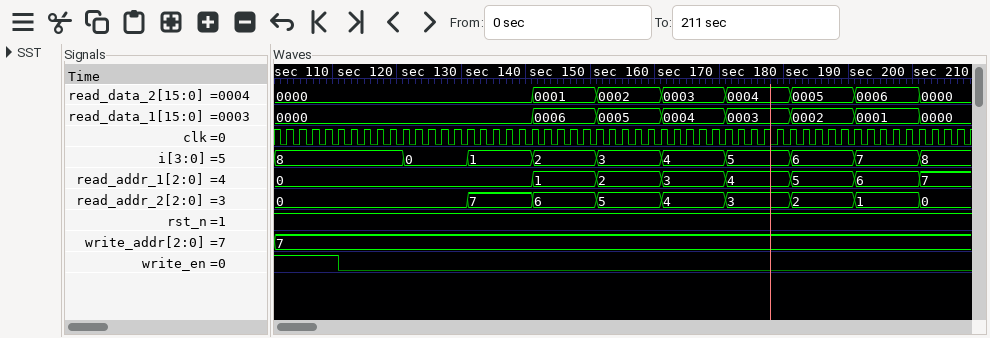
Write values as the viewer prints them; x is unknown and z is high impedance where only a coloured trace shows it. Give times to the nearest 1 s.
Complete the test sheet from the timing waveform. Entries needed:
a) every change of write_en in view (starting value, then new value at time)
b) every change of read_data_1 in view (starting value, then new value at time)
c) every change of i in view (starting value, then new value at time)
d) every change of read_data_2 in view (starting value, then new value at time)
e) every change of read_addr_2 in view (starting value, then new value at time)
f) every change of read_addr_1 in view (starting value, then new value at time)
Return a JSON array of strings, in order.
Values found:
["1, 0 at 111 s", "0000, 0006 at 141 s, 0005 at 151 s, 0004 at 161 s, 0003 at 171 s, 0002 at 181 s, 0001 at 191 s, 0000 at 201 s", "8, 0 at 121 s, 1 at 131 s, 2 at 141 s, 3 at 151 s, 4 at 161 s, 5 at 171 s, 6 at 181 s, 7 at 191 s, 8 at 201 s", "0000, 0001 at 141 s, 0002 at 151 s, 0003 at 161 s, 0004 at 171 s, 0005 at 181 s, 0006 at 191 s, 0000 at 201 s", "0, 7 at 131 s, 6 at 141 s, 5 at 151 s, 4 at 161 s, 3 at 171 s, 2 at 181 s, 1 at 191 s, 0 at 201 s", "0, 1 at 141 s, 2 at 151 s, 3 at 161 s, 4 at 171 s, 5 at 181 s, 6 at 191 s, 7 at 201 s"]
